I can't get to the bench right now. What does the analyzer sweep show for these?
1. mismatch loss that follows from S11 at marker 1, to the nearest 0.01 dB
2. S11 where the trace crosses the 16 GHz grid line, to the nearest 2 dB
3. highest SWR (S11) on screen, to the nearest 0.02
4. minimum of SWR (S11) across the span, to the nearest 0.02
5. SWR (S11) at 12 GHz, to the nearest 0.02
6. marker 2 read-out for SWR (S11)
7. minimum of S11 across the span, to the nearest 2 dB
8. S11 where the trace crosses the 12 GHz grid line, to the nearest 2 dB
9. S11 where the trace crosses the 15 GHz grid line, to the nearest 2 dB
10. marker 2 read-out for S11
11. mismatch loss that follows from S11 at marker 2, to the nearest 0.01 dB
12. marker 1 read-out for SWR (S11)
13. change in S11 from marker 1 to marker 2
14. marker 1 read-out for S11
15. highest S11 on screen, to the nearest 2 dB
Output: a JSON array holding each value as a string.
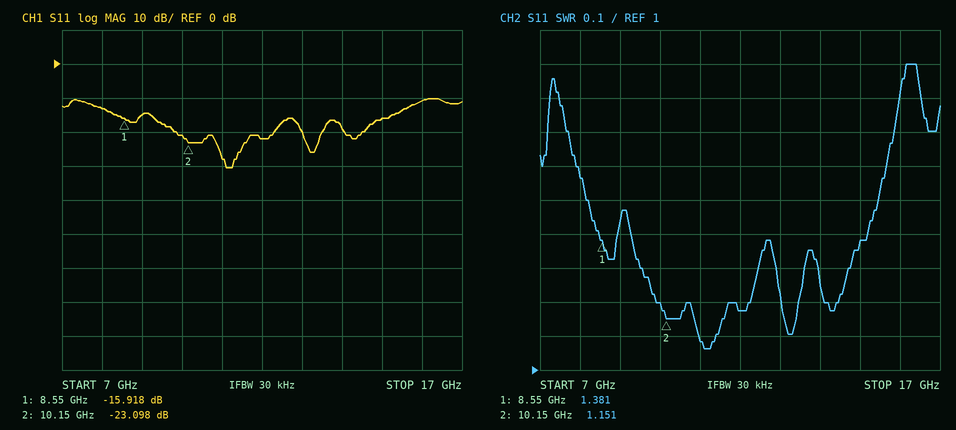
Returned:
["0.11 dB", "-10 dB", "1.90", "1.06", "1.18", "1.151", "-30 dB", "-22 dB", "-16 dB", "-23.098 dB", "0.02 dB", "1.381", "-7.180 dB", "-15.918 dB", "-10 dB"]
